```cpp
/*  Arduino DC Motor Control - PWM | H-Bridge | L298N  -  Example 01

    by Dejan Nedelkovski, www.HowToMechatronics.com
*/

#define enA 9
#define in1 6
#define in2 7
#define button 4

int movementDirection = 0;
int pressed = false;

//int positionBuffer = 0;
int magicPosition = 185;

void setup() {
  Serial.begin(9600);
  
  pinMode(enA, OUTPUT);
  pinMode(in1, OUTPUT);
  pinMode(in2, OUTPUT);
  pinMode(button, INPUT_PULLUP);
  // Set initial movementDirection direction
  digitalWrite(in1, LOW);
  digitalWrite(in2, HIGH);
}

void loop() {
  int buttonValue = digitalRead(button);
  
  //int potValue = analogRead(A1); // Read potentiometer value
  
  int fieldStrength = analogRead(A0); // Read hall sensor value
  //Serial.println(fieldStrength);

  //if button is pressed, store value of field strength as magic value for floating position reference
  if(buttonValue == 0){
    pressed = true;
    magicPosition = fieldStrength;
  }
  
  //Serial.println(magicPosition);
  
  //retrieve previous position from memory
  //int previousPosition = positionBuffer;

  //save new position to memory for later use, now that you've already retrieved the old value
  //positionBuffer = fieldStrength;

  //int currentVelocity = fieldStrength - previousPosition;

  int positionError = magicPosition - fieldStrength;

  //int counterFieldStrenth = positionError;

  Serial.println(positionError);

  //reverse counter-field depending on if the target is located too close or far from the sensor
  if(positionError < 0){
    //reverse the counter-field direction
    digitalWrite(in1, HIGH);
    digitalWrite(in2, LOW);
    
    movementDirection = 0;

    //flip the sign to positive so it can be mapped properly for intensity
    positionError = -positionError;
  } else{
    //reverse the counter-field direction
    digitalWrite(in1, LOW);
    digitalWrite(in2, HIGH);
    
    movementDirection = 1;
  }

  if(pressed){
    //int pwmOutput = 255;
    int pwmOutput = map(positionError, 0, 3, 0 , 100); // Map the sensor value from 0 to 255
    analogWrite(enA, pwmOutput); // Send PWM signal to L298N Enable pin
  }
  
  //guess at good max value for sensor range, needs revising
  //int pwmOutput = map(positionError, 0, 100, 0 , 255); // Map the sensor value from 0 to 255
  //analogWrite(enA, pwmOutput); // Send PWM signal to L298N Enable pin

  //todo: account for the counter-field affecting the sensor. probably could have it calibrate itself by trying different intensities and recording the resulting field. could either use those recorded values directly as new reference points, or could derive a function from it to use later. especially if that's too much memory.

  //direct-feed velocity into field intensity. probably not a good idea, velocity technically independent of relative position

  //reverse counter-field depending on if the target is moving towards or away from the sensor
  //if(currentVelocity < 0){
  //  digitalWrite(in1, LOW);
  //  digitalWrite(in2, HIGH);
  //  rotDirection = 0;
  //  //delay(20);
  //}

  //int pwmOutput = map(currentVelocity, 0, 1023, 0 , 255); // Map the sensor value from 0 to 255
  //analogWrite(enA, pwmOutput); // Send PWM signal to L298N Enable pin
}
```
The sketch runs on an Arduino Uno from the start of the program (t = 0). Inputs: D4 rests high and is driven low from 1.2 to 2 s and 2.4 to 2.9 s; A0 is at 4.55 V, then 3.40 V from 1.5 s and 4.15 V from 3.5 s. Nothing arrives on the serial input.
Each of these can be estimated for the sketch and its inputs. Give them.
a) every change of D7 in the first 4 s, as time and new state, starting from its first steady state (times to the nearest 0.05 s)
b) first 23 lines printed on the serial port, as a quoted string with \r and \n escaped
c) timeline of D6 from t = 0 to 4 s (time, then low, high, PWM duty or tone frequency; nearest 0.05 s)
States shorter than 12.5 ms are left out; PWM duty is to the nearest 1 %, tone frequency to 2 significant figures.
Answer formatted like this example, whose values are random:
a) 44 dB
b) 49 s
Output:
a) 0 s low; 1.2 s high; 3.5 s low
b) "-746\r\n-746\r\n-746\r\n-746\r\n-746\r\n-746\r\n-746\r\n-746\r\n-746\r\n-746\r\n-746\r\n-746\r\n-746\r\n-746\r\n-746\r\n-746\r\n-746\r\n-746\r\n-746\r\n-746\r\n-746\r\n-746\r\n-746\r\n"
c) 0 s high; 1.2 s low; 3.5 s high
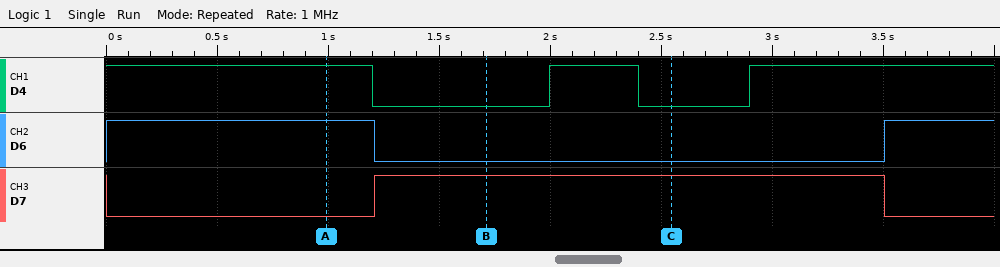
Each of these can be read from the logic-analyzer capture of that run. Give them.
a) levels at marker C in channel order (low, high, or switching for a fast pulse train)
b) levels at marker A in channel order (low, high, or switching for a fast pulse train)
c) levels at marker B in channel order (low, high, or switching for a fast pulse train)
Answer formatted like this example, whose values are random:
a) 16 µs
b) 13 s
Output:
a) D4 low, D6 low, D7 high
b) D4 high, D6 high, D7 low
c) D4 low, D6 low, D7 high
